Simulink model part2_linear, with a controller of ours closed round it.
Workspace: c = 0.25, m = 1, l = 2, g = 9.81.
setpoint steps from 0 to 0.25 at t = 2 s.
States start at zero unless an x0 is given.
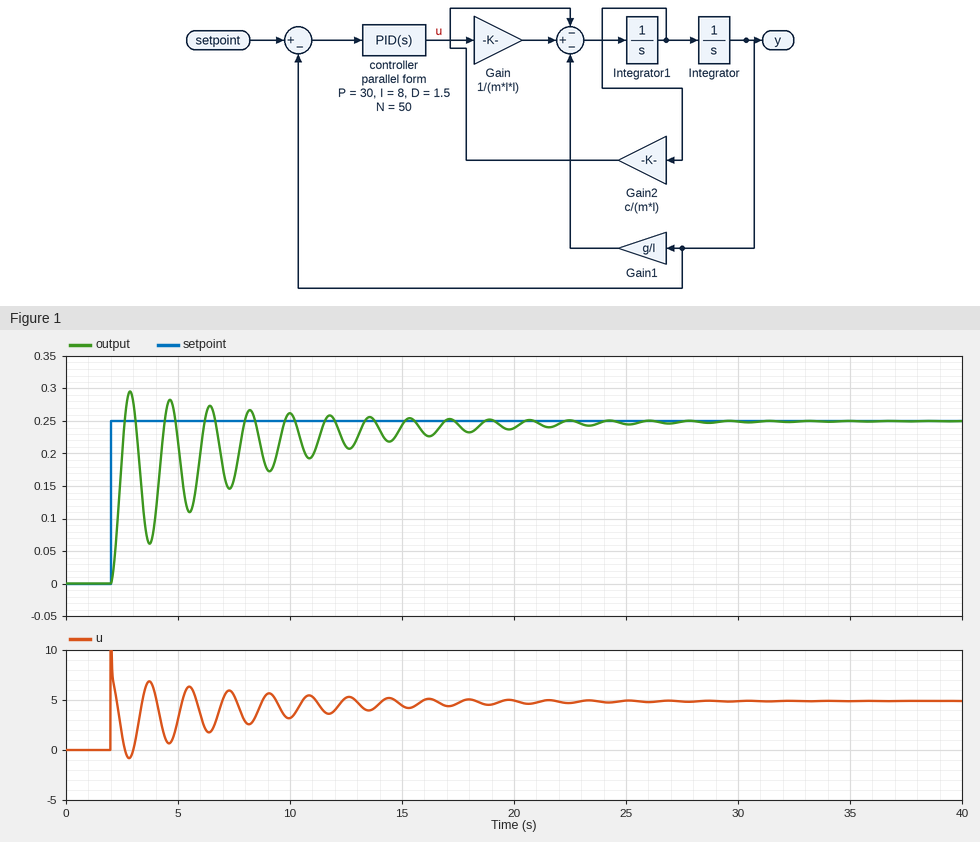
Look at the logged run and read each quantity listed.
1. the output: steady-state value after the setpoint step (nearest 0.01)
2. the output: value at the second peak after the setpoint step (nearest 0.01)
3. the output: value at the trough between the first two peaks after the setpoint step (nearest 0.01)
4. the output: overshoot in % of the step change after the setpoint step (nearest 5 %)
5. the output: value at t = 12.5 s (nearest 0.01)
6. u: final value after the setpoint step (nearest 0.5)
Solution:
0.25
0.28
0.06
20 %
0.21
5.0
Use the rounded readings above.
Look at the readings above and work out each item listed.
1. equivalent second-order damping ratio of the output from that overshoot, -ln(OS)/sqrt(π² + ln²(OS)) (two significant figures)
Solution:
0.46
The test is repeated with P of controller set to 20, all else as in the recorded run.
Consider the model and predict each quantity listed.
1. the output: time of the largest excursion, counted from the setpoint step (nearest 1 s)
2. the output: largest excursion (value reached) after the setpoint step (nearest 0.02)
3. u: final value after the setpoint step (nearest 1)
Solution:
5 s
0.26
5
